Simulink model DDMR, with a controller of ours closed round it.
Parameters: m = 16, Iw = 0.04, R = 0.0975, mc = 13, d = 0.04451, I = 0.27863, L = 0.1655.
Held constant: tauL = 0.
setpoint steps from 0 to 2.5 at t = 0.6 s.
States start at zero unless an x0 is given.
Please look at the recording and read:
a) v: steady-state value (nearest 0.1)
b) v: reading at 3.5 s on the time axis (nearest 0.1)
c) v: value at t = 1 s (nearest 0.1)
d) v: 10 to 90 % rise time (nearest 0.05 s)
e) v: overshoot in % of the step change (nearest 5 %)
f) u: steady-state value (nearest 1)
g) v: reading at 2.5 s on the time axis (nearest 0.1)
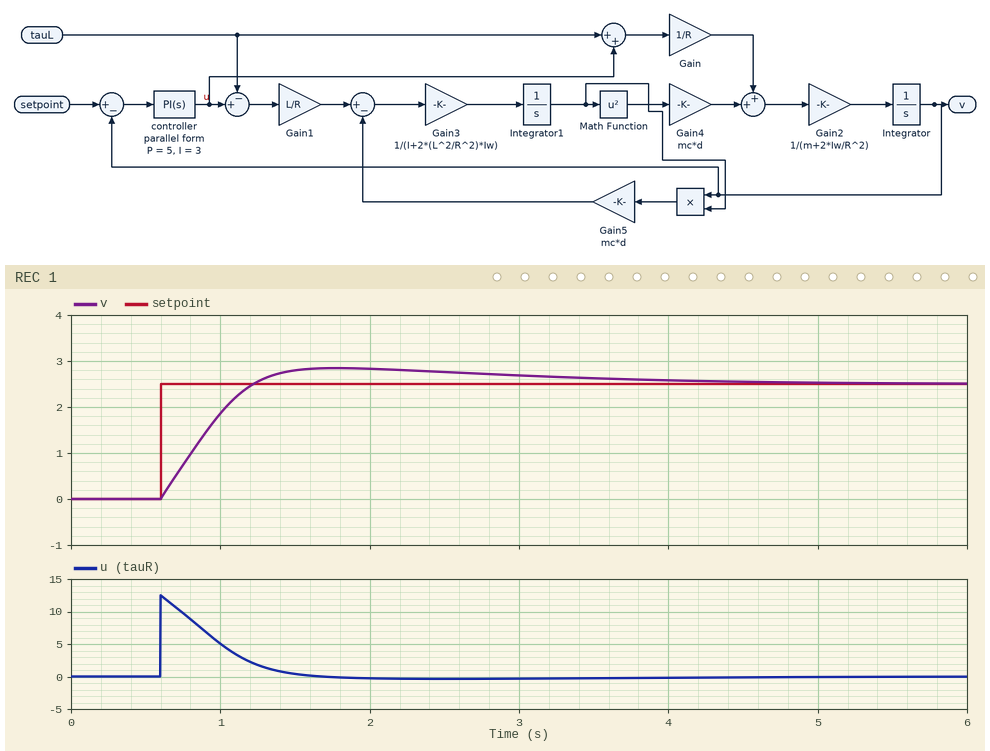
2.5
2.6
1.9
0.45 s
15 %
0
2.8
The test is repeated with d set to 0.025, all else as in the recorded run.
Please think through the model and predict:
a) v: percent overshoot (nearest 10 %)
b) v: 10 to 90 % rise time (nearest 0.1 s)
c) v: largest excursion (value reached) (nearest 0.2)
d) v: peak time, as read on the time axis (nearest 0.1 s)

20 %
0.5 s
3.0
1.8 s
